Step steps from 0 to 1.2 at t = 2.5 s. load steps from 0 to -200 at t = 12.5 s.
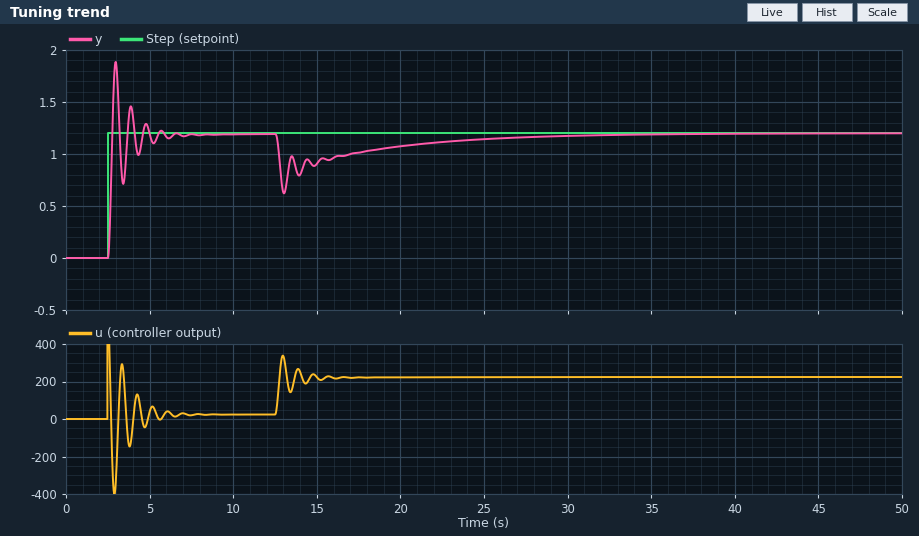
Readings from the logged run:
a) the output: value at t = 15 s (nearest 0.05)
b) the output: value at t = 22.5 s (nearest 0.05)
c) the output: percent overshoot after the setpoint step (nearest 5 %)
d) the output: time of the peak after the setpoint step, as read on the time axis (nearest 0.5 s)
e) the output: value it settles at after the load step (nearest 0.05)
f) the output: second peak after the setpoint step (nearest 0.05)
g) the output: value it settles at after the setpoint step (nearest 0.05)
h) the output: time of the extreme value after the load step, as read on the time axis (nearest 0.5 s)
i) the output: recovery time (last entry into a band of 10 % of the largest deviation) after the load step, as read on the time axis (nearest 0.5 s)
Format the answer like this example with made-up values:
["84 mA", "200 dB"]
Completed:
["0.90", "1.10", "55 %", "3.0 s", "1.20", "1.45", "1.20", "13.0 s", "25.0 s"]
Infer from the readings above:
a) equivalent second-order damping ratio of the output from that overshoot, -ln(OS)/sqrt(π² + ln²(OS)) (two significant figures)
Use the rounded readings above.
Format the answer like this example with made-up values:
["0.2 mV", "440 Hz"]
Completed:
["0.19"]
